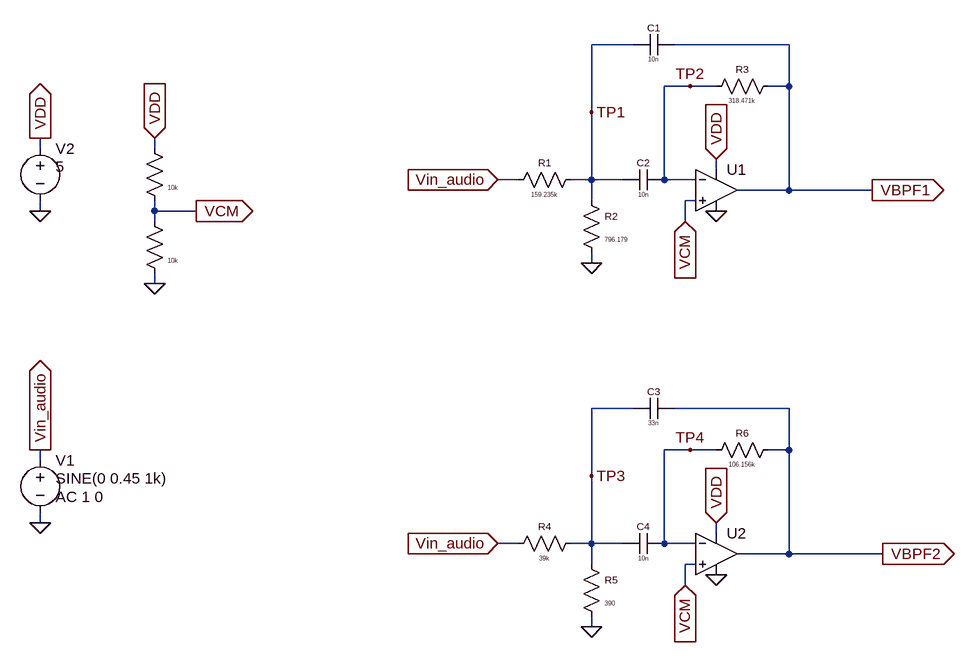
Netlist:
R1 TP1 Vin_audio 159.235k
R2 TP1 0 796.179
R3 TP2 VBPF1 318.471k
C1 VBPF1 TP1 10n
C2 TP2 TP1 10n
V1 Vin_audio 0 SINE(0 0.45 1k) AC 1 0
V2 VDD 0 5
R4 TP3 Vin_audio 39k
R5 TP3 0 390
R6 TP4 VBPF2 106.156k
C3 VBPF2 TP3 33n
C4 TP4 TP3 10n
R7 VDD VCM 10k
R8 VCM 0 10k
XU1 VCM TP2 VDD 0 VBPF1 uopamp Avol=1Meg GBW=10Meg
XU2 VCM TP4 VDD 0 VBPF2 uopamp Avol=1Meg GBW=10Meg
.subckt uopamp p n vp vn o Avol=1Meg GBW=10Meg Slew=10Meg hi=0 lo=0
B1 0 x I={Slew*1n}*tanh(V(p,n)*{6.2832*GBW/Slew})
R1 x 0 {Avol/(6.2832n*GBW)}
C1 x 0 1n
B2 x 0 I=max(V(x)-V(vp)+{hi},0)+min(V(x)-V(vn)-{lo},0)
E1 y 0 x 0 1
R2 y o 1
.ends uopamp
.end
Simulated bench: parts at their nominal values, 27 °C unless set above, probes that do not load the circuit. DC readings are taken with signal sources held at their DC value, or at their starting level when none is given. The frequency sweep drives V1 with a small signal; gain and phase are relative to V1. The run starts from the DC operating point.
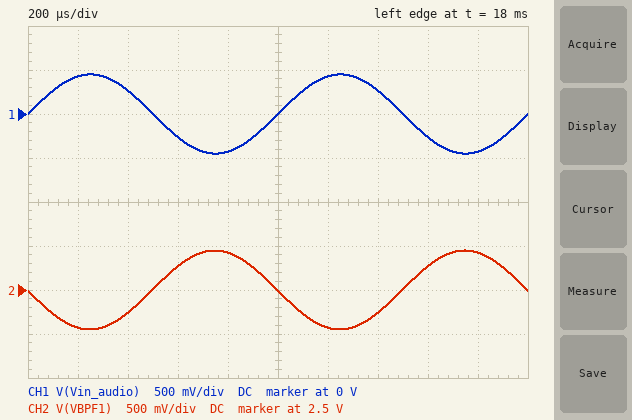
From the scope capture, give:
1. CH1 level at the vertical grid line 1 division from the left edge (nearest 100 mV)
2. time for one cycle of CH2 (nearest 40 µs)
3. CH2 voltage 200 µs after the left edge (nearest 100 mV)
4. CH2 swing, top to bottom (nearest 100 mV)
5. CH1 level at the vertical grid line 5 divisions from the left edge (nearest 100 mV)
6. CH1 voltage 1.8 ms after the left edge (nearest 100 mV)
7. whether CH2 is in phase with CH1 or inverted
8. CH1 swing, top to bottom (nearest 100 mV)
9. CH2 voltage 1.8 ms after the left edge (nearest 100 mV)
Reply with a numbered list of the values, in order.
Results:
1. 400 mV
2. 1.00 ms
3. 2.1 V
4. 900 mV
5. 0 V
6. -400 mV
7. inverted
8. 900 mV
9. 2.9 V
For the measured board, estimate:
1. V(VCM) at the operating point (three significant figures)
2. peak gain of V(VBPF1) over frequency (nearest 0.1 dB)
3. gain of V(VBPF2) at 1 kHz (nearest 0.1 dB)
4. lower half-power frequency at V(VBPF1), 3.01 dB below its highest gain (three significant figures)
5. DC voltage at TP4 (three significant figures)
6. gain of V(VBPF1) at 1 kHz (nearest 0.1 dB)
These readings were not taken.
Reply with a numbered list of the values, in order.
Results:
1. 2.50 V
2. 0 dB
3. -17.2 dB
4. 952 Hz
5. 2.50 V
6. 0 dB
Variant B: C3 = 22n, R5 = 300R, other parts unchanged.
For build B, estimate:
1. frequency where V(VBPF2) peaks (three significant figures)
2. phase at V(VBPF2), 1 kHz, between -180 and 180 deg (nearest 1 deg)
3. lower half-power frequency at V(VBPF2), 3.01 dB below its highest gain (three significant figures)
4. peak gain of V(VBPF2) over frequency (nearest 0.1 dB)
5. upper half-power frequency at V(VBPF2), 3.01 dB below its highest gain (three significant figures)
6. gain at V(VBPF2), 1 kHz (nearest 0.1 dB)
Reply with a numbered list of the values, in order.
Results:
1. 1.91 kHz
2. -95 deg
3. 1.80 kHz
4. -1.4 dB
5. 2.02 kHz
6. -23.1 dB
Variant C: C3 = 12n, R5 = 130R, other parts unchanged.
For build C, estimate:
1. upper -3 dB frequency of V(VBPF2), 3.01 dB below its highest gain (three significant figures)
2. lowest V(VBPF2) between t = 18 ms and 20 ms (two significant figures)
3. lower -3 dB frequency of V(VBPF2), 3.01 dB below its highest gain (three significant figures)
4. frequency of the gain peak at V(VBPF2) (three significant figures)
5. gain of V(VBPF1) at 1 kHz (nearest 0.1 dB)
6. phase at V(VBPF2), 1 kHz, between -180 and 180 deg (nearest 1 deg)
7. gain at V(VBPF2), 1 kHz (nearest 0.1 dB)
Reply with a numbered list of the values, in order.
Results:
1. 4.04 kHz
2. 2.5 V
3. 3.76 kHz
4. 3.90 kHz
5. 0 dB
6. -91 deg
7. -32.5 dB
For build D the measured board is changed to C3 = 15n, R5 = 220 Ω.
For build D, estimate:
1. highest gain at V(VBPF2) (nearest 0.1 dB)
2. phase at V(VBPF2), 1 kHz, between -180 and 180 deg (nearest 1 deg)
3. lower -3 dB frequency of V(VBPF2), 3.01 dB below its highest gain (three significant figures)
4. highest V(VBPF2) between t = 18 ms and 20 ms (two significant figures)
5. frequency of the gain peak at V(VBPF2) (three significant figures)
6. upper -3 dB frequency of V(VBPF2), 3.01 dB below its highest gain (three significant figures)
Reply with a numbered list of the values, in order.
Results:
1. 0.7 dB
2. -92 deg
3. 2.57 kHz
4. 2.5 V
5. 2.69 kHz
6. 2.82 kHz
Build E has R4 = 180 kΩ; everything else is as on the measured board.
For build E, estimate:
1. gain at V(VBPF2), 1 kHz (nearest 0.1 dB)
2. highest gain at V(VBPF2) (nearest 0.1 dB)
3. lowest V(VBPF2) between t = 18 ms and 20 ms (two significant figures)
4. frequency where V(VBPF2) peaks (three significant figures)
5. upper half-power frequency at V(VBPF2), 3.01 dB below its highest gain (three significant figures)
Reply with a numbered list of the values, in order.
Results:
1. -30.3 dB
2. -17.3 dB
3. 2.5 V
4. 1.36 kHz
5. 1.46 kHz
